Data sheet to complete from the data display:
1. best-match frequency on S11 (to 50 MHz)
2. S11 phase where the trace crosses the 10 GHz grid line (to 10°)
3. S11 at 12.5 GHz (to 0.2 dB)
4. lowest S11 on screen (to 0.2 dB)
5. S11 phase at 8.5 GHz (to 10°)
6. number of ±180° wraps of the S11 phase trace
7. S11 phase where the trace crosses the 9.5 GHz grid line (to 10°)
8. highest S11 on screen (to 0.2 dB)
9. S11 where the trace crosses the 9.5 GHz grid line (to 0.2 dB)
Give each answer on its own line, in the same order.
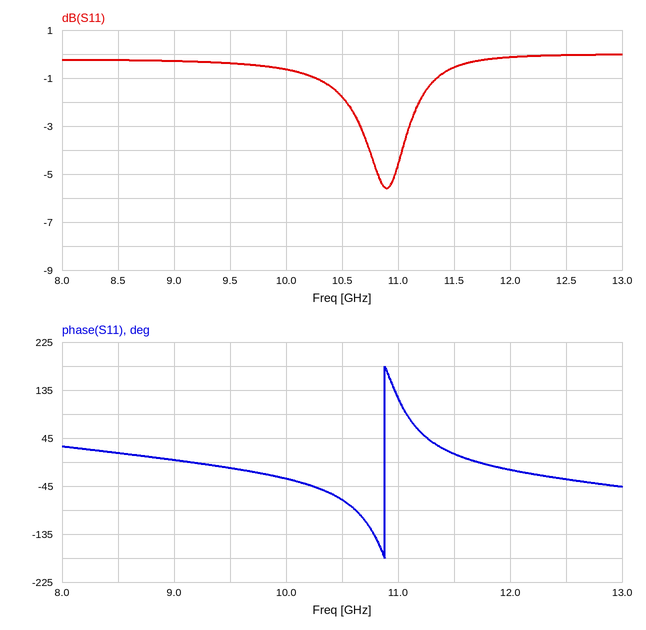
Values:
10.90 GHz
-30°
0.0 dB
-5.6 dB
20°
1
-10°
0.0 dB
-0.4 dB
